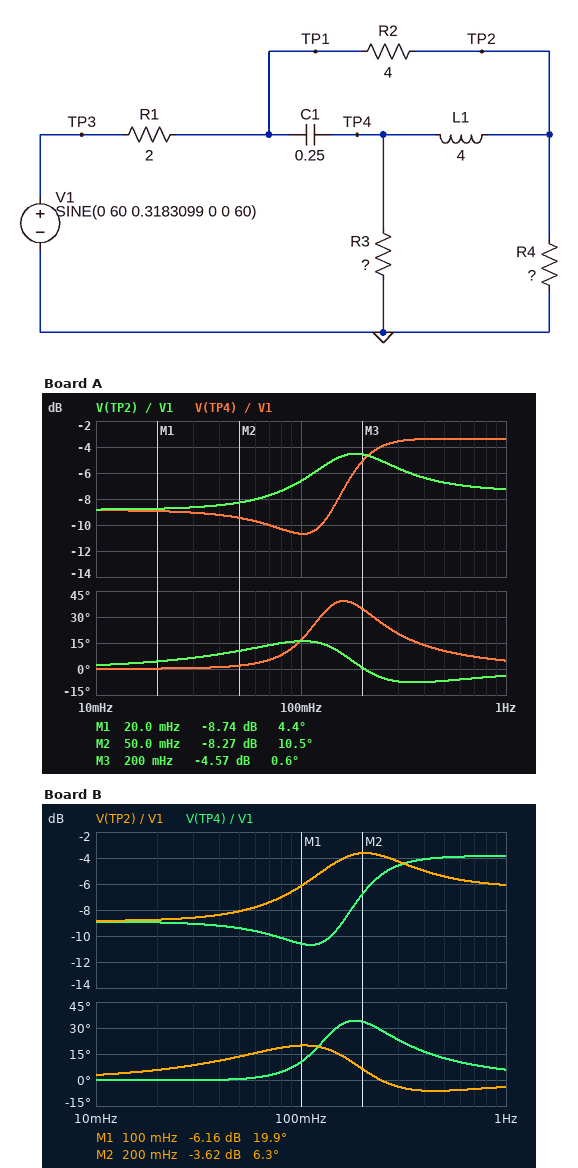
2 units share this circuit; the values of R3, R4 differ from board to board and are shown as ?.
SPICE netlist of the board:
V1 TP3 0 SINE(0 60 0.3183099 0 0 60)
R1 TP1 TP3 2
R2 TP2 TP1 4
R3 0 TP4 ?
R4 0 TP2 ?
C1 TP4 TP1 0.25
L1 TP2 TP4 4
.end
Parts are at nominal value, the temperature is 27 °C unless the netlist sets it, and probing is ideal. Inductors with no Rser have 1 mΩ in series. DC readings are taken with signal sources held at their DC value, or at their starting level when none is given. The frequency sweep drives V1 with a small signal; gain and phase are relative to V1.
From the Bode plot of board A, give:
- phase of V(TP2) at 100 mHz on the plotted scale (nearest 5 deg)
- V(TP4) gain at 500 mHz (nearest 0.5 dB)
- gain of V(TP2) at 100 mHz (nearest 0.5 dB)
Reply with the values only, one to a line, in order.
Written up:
15 deg
-3.5 dB
-6.5 dB
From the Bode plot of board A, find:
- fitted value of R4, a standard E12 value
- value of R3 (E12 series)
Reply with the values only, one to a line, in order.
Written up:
6.8 Ω
6.8 Ω
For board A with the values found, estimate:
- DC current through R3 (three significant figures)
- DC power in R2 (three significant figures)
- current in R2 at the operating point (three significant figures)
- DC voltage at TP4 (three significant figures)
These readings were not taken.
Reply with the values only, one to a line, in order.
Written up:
2.76 A
122 W
5.53 A
18.8 V
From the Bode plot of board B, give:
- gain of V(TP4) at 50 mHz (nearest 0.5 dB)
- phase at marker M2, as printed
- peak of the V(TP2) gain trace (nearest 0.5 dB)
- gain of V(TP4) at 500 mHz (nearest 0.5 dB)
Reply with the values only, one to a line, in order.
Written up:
-9.5 dB
6.3 deg
-3.5 dB
-4.0 dB
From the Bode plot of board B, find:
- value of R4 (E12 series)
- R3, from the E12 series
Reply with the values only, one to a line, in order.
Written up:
12 Ω
4.7 Ω
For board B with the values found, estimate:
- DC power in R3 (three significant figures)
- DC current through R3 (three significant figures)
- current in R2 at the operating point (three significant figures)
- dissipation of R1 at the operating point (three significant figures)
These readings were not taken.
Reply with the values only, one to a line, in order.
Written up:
74.5 W
3.98 A
5.54 A
61.4 W
